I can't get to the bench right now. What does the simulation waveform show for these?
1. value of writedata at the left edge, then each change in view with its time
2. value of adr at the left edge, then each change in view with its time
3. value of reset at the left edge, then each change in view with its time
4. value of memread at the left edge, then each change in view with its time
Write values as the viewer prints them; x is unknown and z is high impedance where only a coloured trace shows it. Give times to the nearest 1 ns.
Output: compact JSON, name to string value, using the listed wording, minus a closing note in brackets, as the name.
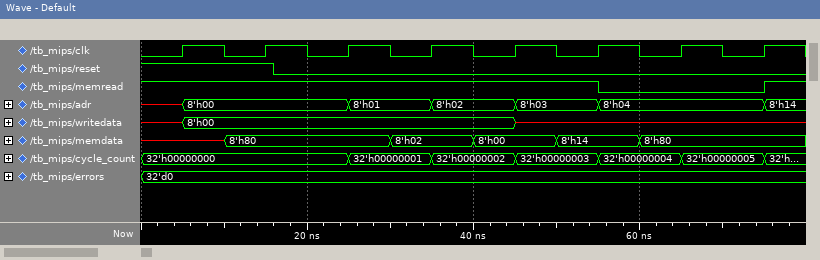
{"value of writedata at the left edge, then each change in view with its time": "x, 8'h00 at 5 ns, x at 45 ns", "value of adr at the left edge, then each change in view with its time": "x, 8'h00 at 5 ns, 8'h01 at 25 ns, 8'h02 at 35 ns, 8'h03 at 45 ns, 8'h04 at 55 ns, 8'h14 at 75 ns", "value of reset at the left edge, then each change in view with its time": "1, 0 at 16 ns", "value of memread at the left edge, then each change in view with its time": "1, 0 at 55 ns, 1 at 75 ns"}
